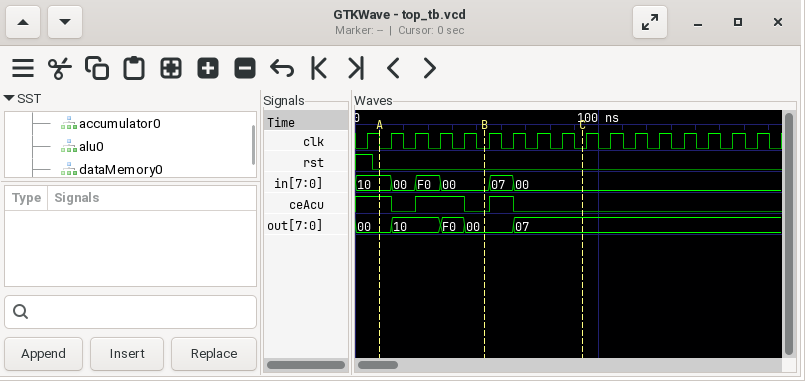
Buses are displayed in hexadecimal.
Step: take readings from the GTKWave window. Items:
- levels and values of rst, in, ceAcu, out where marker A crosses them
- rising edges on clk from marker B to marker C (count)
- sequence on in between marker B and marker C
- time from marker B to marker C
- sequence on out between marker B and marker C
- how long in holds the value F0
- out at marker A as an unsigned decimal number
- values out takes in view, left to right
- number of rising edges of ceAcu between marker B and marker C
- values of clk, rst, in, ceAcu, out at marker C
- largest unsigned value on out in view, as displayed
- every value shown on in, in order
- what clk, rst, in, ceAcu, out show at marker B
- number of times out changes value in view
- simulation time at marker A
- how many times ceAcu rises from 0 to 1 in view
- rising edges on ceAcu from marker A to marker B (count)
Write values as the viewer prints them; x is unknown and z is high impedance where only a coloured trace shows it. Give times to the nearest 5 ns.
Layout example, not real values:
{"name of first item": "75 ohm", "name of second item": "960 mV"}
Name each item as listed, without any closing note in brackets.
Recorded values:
{"levels and values of rst, in, ceAcu, out where marker A crosses them": "rst=0, in=10, ceAcu=1, out=00", "rising edges on clk from marker B to marker C": "4", "sequence on in between marker B and marker C": "00, 07, 00", "time from marker B to marker C": "40 ns", "sequence on out between marker B and marker C": "00, 07", "how long in holds the value F0": "10 ns", "out at marker A as an unsigned decimal number": "0", "values out takes in view, left to right": "00, 10, F0, 00, 07", "number of rising edges of ceAcu between marker B and marker C": "1", "values of clk, rst, in, ceAcu, out at marker C": "clk=0, rst=0, in=00, ceAcu=0, out=07", "largest unsigned value on out in view, as displayed": "F0", "every value shown on in, in order": "10, 00, F0, 00, 07, 00", "what clk, rst, in, ceAcu, out show at marker B": "clk=0, rst=0, in=00, ceAcu=0, out=00", "number of times out changes value in view": "4", "simulation time at marker A": "10 ns", "how many times ceAcu rises from 0 to 1 in view": "2", "rising edges on ceAcu from marker A to marker B": "1"}
